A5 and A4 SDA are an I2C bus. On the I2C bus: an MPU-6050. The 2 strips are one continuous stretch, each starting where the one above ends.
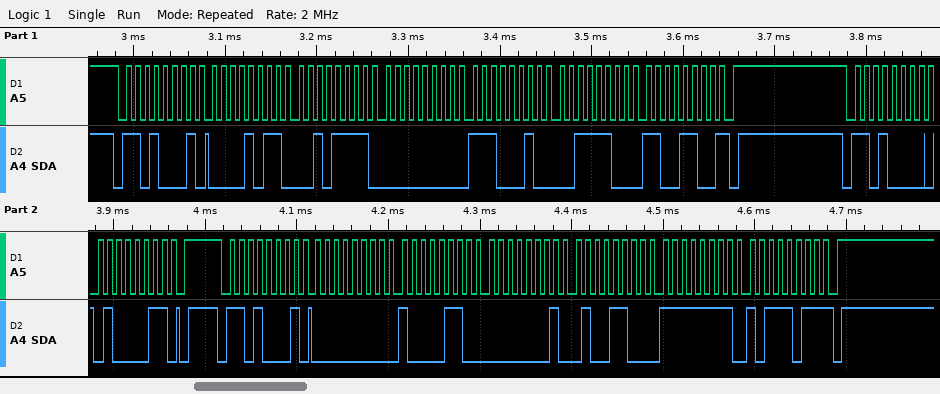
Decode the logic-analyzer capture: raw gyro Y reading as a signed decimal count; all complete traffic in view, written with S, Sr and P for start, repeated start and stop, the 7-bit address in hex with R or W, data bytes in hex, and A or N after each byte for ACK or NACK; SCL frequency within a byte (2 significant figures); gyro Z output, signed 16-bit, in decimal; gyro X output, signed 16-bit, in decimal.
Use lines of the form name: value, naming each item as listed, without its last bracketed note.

raw gyro Y reading as a signed decimal count: 332
all complete traffic in view, written with S, Sr and P for start, repeated start and stop, the 7-bit address in hex with R or W, data bytes in hex, and A or N after each byte for ACK or NACK: S 68R A 0B A 2F A 00 A E2 A 3C A CC N P S 68W A 43 A P S 68R A 00 A 86 A 01 A 4C A FF A BB N P
SCL frequency within a byte: 100 kHz
gyro Z output, signed 16-bit, in decimal: -69
gyro X output, signed 16-bit, in decimal: 134
